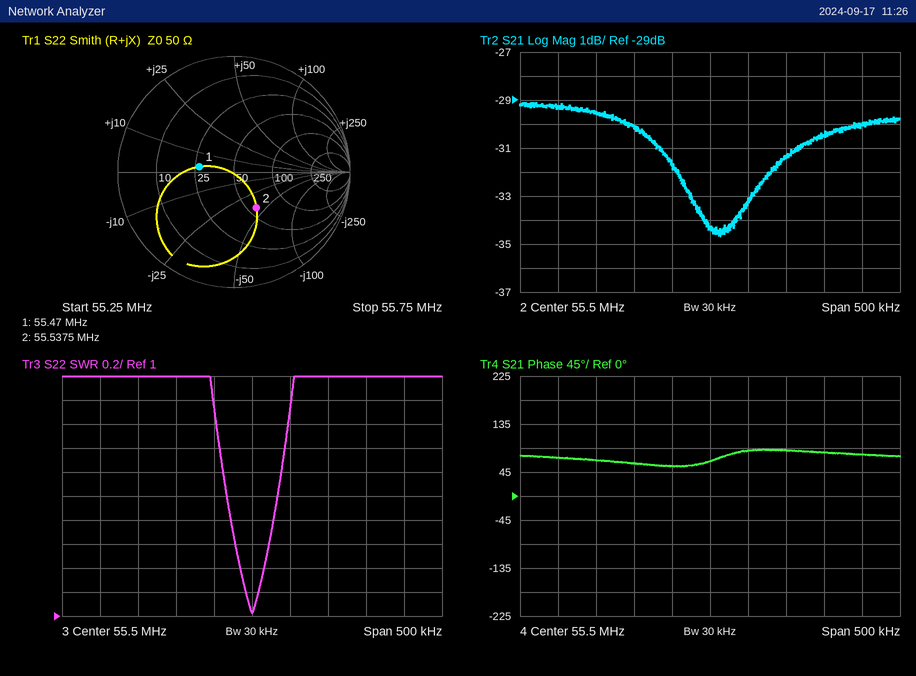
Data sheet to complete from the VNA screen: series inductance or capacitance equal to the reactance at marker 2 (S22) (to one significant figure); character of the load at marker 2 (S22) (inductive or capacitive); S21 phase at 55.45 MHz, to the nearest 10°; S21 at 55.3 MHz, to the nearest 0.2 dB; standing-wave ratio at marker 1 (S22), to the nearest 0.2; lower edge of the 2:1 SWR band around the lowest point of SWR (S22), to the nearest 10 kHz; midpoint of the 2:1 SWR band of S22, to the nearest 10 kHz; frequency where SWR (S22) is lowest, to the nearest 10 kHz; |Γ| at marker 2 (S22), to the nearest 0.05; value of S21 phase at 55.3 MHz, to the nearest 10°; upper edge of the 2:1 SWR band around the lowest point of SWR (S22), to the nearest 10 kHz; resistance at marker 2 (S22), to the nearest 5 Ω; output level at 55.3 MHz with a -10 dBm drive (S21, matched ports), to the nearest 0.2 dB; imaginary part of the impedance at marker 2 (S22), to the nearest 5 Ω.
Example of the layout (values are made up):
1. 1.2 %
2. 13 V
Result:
1. 70 pF
2. capacitive
3. 60°
4. -29.2 dB
5. 1.8
6. 55.47 MHz
7. 55.50 MHz
8. 55.50 MHz
9. 0.35
10. 70°
11. 55.53 MHz
12. 60 Ω
13. -39.2 dBm
14. -40 Ω
